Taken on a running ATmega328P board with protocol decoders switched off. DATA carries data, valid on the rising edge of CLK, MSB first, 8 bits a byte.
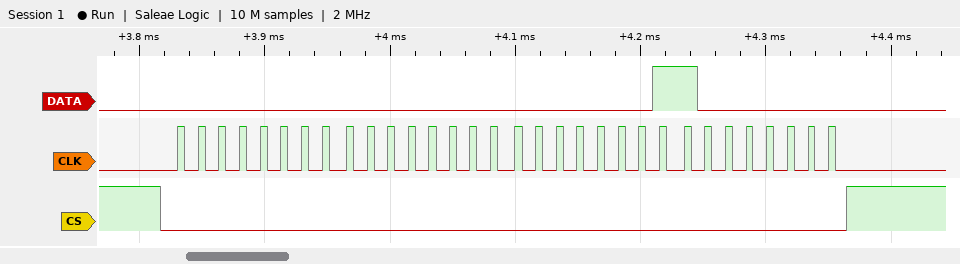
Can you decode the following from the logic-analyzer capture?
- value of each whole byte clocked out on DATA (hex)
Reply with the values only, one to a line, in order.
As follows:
0x00 0x00 0x01 0x80
